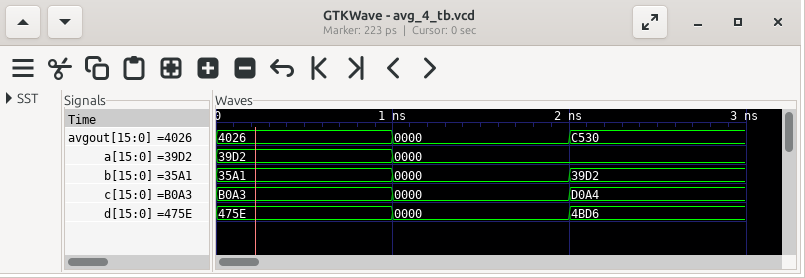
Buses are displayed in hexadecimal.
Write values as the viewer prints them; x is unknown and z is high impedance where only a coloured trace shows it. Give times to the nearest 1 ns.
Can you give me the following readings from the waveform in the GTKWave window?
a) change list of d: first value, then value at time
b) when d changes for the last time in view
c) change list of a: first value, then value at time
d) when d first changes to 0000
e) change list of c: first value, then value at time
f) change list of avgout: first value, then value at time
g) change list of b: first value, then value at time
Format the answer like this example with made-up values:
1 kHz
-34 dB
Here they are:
475E, 0000 at 1 ns, 4BD6 at 2 ns
2 ns
39D2, 0000 at 1 ns
1 ns
B0A3, 0000 at 1 ns, D0A4 at 2 ns
4026, 0000 at 1 ns, C530 at 2 ns
35A1, 0000 at 1 ns, 39D2 at 2 ns
